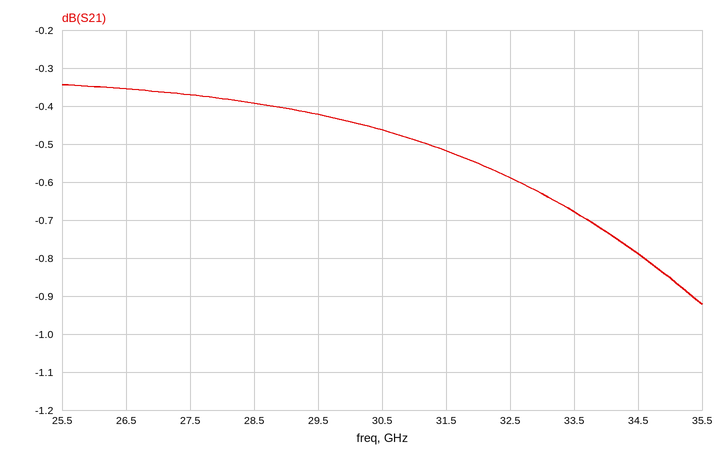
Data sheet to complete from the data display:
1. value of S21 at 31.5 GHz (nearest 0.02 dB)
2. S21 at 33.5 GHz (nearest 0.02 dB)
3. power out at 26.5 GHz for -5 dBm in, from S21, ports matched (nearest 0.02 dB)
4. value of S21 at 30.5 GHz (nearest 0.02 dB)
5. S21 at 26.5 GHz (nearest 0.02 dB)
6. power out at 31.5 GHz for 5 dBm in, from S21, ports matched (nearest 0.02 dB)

-0.52 dB
-0.68 dB
-5.36 dBm
-0.46 dB
-0.36 dB
4.48 dBm
